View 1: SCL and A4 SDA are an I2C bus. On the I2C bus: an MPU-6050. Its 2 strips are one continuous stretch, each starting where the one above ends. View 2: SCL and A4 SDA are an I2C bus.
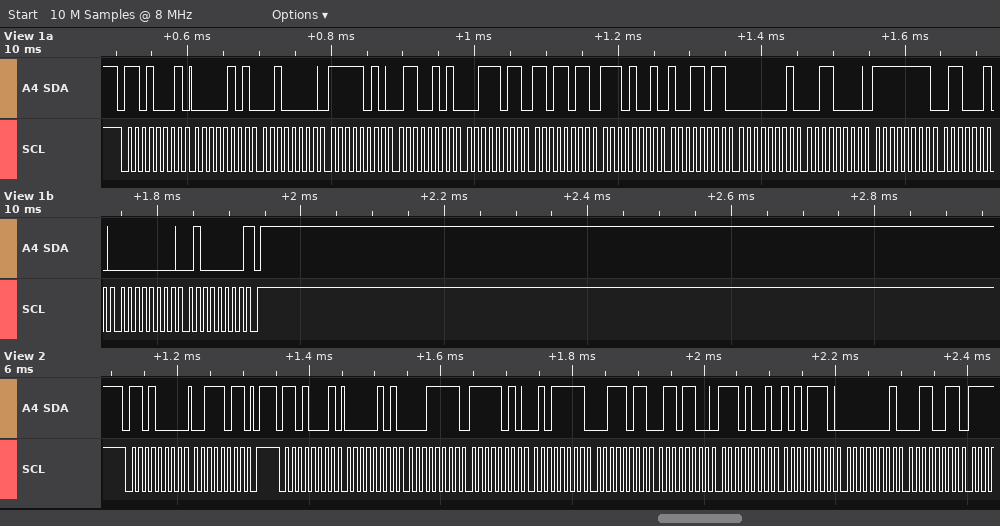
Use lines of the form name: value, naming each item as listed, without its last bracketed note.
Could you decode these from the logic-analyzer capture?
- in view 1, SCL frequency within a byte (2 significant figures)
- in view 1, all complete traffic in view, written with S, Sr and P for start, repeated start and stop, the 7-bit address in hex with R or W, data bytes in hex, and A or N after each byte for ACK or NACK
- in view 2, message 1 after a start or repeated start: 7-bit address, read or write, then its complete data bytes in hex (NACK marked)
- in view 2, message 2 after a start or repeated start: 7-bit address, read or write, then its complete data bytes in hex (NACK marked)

in view 1, SCL frequency within a byte: 100 kHz
in view 1, all complete traffic in view, written with S, Sr and P for start, repeated start and stop, the 7-bit address in hex with R or W, data bytes in hex, and A or N after each byte for ACK or NACK: S 68R A 05 A 20 A FA A 65 A 3B A DB A E9 A 9B A 01 A 30 A FF A 62 A 00 A 40 N P
in view 2, message 1 after a start or repeated start: 7-bit address, read or write, then its complete data bytes in hex: 0x68 write: 3B
in view 2, message 2 after a start or repeated start: 7-bit address, read or write, then its complete data bytes in hex: 0x68 read: 05 1F FA 5F 3B 6C E9 AE 01 33
